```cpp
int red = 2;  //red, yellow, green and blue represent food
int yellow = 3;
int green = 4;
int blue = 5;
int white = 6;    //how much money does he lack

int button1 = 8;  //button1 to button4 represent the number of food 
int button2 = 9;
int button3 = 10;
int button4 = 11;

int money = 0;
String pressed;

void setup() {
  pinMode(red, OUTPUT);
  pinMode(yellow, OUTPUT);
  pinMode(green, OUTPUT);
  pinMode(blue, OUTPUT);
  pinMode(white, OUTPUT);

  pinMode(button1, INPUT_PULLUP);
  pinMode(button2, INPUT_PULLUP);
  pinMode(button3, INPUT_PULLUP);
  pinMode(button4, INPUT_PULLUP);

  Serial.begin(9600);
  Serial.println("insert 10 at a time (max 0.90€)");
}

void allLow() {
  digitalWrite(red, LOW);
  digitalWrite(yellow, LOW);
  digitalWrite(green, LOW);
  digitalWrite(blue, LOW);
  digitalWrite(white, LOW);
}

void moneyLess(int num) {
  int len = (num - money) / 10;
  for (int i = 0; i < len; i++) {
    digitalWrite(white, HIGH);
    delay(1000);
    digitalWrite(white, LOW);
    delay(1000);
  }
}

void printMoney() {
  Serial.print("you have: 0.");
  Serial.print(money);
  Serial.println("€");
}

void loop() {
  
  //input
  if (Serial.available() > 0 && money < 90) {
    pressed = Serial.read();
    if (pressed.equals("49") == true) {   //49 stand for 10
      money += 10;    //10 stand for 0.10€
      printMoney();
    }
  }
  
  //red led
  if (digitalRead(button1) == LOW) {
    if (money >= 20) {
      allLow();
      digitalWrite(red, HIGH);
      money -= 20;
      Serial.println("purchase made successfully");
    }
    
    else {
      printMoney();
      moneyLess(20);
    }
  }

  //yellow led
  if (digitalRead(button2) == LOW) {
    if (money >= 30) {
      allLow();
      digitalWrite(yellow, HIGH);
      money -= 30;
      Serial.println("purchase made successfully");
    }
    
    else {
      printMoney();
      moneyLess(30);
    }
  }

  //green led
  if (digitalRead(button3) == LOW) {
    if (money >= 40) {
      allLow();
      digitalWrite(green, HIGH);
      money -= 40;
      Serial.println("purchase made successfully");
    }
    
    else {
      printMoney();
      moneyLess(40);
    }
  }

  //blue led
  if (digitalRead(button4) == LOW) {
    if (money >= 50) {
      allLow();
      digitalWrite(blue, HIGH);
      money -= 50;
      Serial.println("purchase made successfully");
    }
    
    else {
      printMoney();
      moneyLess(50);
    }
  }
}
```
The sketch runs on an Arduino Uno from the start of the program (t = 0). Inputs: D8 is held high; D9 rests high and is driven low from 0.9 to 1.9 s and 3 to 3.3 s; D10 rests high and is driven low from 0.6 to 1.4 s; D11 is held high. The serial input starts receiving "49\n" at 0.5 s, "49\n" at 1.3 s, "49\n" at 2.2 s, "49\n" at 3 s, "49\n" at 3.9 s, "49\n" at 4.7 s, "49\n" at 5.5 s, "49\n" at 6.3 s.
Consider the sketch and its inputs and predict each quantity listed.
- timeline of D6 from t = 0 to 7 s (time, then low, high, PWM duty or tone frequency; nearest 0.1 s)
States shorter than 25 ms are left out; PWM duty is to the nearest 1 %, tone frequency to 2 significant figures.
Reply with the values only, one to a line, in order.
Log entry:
0 s low; 0.6 s high; 1.6 s low; 2.6 s high; 3.6 s low; 4.6 s high; 5.6 s low; 6.6 s high
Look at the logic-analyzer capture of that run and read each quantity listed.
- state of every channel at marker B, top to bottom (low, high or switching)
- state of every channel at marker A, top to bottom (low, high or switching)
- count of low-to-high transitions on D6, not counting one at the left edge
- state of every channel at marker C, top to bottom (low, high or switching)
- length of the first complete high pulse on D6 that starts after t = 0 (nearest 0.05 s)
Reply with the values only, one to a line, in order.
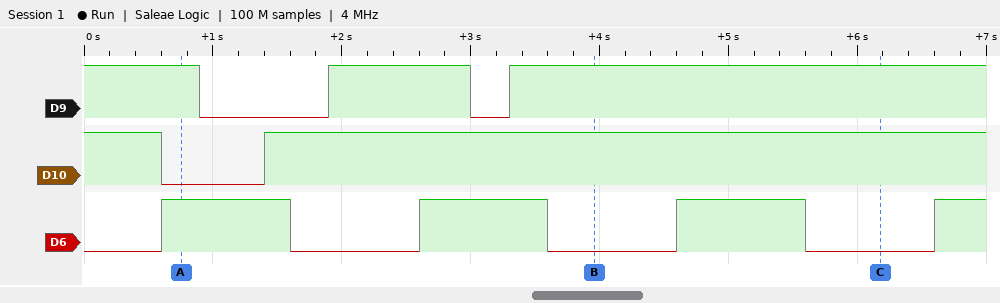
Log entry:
D9 high, D10 high, D6 low
D9 high, D10 low, D6 high
4
D9 high, D10 high, D6 low
1.00 s
